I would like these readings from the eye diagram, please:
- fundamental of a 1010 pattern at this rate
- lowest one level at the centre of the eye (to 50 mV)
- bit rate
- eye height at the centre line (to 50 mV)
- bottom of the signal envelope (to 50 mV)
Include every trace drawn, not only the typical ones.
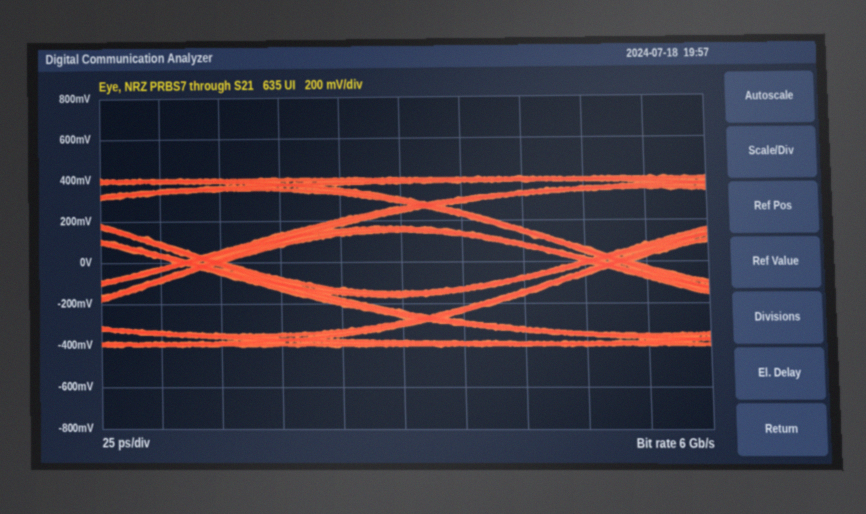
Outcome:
3 GHz
150 mV
6 Gb/s
300 mV
-400 mV
